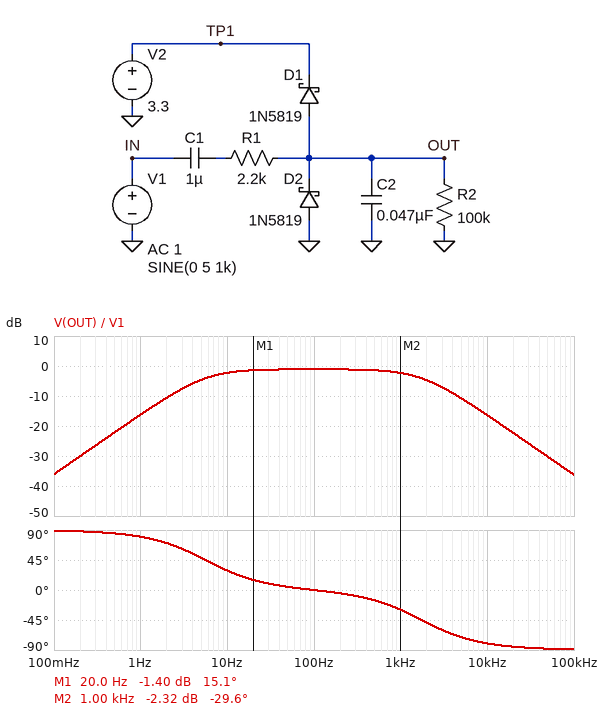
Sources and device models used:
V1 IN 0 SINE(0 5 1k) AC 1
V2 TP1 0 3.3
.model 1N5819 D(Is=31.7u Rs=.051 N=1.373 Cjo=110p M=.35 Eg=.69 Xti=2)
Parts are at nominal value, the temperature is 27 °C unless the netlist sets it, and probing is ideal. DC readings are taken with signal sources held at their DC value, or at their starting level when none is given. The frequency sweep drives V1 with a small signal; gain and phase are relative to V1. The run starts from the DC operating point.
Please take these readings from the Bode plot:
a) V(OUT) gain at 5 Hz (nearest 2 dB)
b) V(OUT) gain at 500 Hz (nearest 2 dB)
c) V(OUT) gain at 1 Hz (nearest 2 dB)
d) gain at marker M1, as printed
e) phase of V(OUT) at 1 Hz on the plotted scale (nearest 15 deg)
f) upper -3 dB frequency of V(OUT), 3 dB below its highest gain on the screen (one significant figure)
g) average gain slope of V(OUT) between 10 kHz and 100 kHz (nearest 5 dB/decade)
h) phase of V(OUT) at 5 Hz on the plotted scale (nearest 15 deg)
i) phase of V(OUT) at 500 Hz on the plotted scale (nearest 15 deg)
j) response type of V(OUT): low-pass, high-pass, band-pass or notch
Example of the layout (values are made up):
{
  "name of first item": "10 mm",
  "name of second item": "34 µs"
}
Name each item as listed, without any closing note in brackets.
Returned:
{
  "V(OUT) gain at 5 Hz": "-4 dB",
  "V(OUT) gain at 500 Hz": "-2 dB",
  "V(OUT) gain at 1 Hz": "-16 dB",
  "gain at marker M1, as printed": "-1.40 dB",
  "phase of V(OUT) at 1 Hz on the plotted scale": "75 deg",
  "upper -3 dB frequency of V(OUT), 3 dB below its highest gain on the screen": "2 kHz",
  "average gain slope of V(OUT) between 10 kHz and 100 kHz": "-20 dB/decade",
  "phase of V(OUT) at 5 Hz on the plotted scale": "45 deg",
  "phase of V(OUT) at 500 Hz on the plotted scale": "-15 deg",
  "response type of V(OUT): low-pass, high-pass, band-pass or notch": "band-pass"
}
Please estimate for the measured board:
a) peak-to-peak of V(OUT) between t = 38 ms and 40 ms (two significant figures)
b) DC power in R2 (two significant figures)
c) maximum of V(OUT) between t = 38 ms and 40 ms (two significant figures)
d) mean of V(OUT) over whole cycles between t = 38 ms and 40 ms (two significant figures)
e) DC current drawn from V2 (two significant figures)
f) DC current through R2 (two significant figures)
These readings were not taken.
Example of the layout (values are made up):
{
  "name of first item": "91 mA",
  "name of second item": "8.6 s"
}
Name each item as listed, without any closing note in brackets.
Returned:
{
  "peak-to-peak of V(OUT) between t = 38 ms and 40 ms": "3.6 V",
  "DC power in R2": "140 nW",
  "maximum of V(OUT) between t = 38 ms and 40 ms": "3.4 V",
  "mean of V(OUT) over whole cycles between t = 38 ms and 40 ms": "1.6 V",
  "DC current drawn from V2": "32 µA",
  "DC current through R2": "1.2 µA"
}
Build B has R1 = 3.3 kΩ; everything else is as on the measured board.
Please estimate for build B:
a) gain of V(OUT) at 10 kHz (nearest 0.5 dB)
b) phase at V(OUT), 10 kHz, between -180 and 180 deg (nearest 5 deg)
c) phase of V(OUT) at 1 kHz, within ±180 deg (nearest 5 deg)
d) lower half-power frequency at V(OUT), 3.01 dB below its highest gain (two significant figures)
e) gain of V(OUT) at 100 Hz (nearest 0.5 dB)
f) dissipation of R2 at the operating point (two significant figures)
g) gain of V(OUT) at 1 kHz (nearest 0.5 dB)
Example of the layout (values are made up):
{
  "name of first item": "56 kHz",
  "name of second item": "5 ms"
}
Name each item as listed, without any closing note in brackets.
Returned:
{
  "gain of V(OUT) at 10 kHz": "-20.0 dB",
  "phase at V(OUT), 10 kHz, between -180 and 180 deg": "-85 deg",
  "phase of V(OUT) at 1 kHz, within ±180 deg": "-40 deg",
  "lower half-power frequency at V(OUT), 3.01 dB below its highest gain": "5.4 Hz",
  "gain of V(OUT) at 100 Hz": "-1.5 dB",
  "dissipation of R2 at the operating point": "140 nW",
  "gain of V(OUT) at 1 kHz": "-3.5 dB"
}
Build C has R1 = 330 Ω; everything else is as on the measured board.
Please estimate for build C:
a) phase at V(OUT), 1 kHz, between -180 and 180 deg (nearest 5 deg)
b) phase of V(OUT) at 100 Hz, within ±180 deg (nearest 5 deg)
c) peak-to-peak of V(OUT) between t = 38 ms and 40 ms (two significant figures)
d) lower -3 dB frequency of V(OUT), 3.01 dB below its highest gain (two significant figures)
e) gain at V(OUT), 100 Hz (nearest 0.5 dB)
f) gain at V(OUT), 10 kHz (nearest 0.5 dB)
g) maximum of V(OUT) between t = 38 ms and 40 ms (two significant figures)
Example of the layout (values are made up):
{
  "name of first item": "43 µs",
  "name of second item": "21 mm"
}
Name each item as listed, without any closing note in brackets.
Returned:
{
  "phase at V(OUT), 1 kHz, between -180 and 180 deg": "-5 deg",
  "phase of V(OUT) at 100 Hz, within ±180 deg": "5 deg",
  "peak-to-peak of V(OUT) between t = 38 ms and 40 ms": "3.7 V",
  "lower -3 dB frequency of V(OUT), 3.01 dB below its highest gain": "6.0 Hz",
  "gain at V(OUT), 100 Hz": "-0.5 dB",
  "gain at V(OUT), 10 kHz": "-3.0 dB",
  "maximum of V(OUT) between t = 38 ms and 40 ms": "3.5 V"
}
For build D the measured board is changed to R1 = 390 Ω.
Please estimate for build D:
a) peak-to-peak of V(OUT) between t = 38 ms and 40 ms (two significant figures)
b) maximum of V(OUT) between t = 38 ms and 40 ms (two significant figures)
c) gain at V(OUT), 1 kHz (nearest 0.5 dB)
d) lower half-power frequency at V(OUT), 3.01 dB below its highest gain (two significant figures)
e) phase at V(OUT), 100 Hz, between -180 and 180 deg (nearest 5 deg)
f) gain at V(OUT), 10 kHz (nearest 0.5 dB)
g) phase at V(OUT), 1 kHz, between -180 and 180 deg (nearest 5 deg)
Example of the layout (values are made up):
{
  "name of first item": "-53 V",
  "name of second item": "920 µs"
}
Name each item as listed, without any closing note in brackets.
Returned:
{
  "peak-to-peak of V(OUT) between t = 38 ms and 40 ms": "3.7 V",
  "maximum of V(OUT) between t = 38 ms and 40 ms": "3.5 V",
  "gain at V(OUT), 1 kHz": "-0.5 dB",
  "lower half-power frequency at V(OUT), 3.01 dB below its highest gain": "6.0 Hz",
  "phase at V(OUT), 100 Hz, between -180 and 180 deg": "5 deg",
  "gain at V(OUT), 10 kHz": "-4.0 dB",
  "phase at V(OUT), 1 kHz, between -180 and 180 deg": "-5 deg"
}
